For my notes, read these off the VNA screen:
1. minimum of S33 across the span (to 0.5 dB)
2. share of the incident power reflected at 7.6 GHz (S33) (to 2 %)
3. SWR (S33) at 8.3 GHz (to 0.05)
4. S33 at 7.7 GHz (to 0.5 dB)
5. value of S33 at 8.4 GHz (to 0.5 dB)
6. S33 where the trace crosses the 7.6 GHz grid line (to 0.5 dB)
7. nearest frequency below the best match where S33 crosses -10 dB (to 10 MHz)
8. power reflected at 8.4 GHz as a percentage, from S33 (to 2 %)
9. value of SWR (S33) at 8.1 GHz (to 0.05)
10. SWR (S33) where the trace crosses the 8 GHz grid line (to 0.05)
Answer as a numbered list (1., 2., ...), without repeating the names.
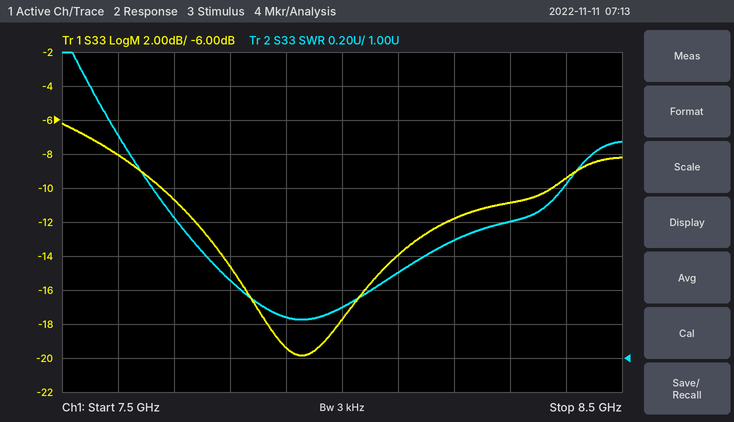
1. -20.0 dB
2. 16 %
3. 1.80
4. -10.5 dB
5. -9.5 dB
6. -8.0 dB
7. 7.68 GHz
8. 12 %
9. 1.50
10. 1.30
